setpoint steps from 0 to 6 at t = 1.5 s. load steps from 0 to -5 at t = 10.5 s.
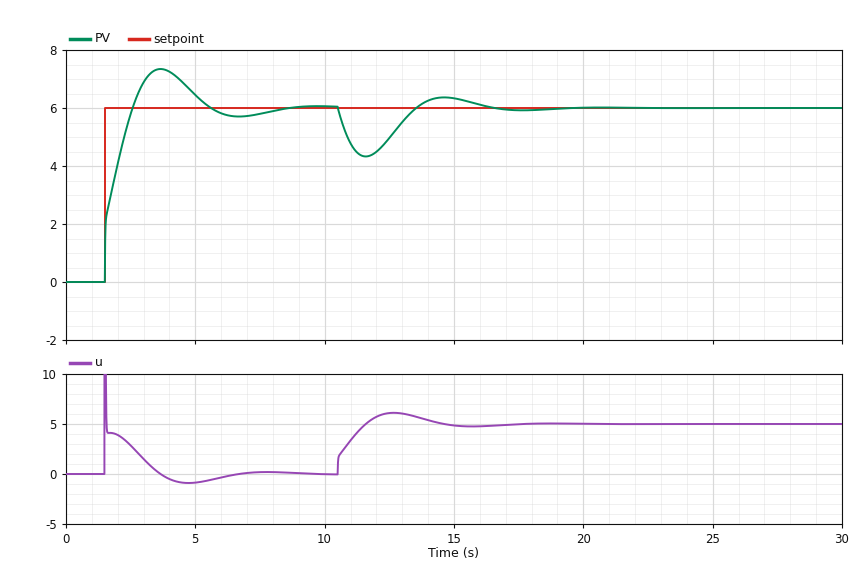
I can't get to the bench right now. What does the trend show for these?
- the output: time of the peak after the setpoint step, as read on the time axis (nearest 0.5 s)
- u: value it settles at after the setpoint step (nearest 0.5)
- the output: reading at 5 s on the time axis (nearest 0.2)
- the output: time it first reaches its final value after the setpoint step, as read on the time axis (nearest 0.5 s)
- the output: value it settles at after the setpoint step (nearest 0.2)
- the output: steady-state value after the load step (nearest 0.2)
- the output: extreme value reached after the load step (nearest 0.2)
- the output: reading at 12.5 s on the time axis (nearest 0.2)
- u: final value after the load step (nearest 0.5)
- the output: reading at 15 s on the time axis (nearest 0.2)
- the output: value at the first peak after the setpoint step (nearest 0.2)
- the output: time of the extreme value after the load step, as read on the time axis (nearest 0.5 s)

3.5 s
0.0
6.4
2.5 s
6.0
6.0
4.4
5.0
5.0
6.4
7.4
11.5 s
